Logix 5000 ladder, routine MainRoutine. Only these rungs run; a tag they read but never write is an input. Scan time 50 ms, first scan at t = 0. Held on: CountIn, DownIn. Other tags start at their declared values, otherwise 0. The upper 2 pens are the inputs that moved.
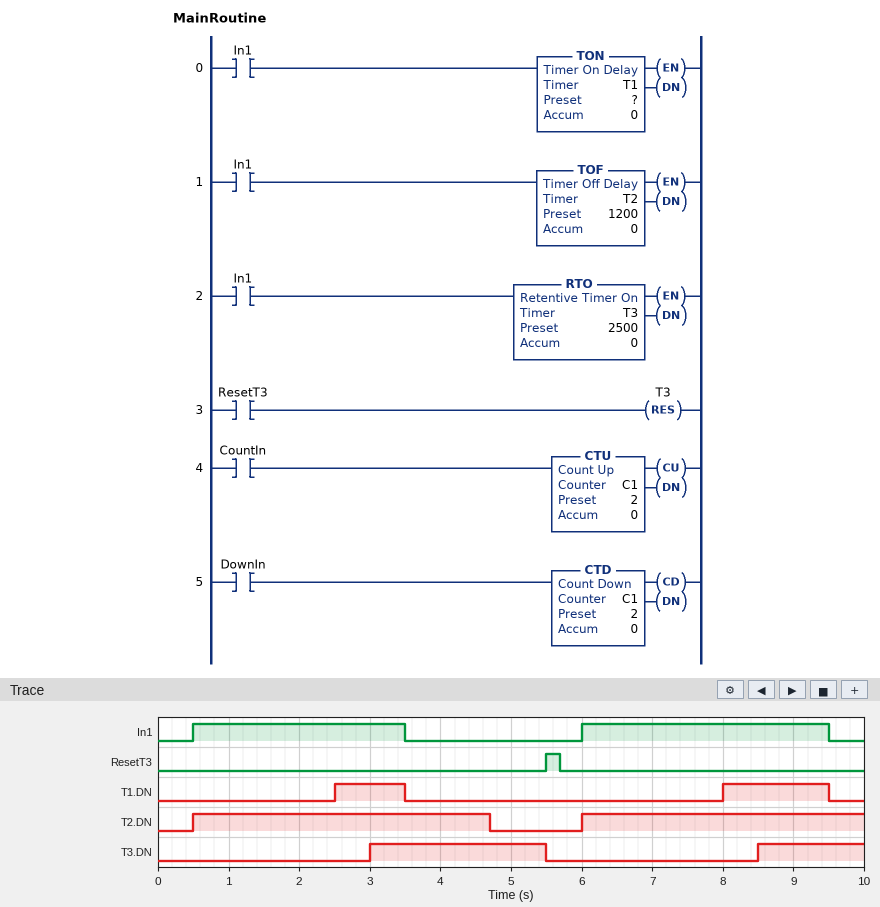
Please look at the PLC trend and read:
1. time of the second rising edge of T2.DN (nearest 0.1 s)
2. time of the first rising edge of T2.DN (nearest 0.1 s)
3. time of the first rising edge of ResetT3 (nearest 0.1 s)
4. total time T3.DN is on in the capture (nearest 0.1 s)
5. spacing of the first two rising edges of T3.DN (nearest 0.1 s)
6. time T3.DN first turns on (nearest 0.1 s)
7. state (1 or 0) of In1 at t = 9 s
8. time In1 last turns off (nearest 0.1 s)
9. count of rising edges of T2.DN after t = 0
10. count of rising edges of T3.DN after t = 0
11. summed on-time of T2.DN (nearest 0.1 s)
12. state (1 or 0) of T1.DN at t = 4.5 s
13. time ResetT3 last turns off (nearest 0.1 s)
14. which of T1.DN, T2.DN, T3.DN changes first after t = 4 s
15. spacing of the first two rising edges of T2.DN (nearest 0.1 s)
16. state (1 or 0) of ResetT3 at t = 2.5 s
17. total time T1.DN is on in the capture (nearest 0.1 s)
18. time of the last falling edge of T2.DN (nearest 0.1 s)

6.0 s
0.5 s
5.5 s
4.0 s
5.5 s
3.0 s
1
9.5 s
2
2
8.2 s
0
5.7 s
T2.DN
5.5 s
0
2.5 s
4.7 s
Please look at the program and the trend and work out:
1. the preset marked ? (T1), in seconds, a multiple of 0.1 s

2.0 s
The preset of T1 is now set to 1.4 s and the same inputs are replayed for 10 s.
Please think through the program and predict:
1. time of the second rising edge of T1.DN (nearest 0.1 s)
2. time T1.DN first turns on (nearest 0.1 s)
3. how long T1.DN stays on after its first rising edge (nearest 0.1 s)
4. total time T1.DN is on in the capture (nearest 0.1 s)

7.4 s
1.9 s
1.6 s
3.7 s
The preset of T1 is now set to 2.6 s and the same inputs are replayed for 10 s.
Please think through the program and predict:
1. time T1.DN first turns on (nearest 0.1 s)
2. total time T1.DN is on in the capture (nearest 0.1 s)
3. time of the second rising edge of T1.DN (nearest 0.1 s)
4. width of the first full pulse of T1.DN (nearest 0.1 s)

3.1 s
1.3 s
8.6 s
0.4 s
